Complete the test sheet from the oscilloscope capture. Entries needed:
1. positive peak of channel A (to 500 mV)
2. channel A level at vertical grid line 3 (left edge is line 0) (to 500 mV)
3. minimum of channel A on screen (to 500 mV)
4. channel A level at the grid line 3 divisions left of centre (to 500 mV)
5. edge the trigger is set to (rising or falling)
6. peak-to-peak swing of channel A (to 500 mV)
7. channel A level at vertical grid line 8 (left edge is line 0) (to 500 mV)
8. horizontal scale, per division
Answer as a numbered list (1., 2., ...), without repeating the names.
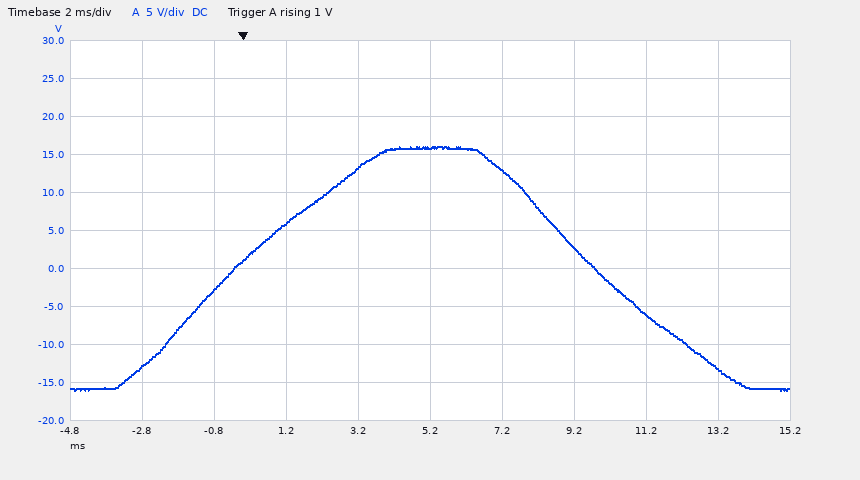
1. 16.0 V
2. 6.0 V
3. -16.0 V
4. -3.0 V
5. rising
6. 32.0 V
7. -6.0 V
8. 2 ms
